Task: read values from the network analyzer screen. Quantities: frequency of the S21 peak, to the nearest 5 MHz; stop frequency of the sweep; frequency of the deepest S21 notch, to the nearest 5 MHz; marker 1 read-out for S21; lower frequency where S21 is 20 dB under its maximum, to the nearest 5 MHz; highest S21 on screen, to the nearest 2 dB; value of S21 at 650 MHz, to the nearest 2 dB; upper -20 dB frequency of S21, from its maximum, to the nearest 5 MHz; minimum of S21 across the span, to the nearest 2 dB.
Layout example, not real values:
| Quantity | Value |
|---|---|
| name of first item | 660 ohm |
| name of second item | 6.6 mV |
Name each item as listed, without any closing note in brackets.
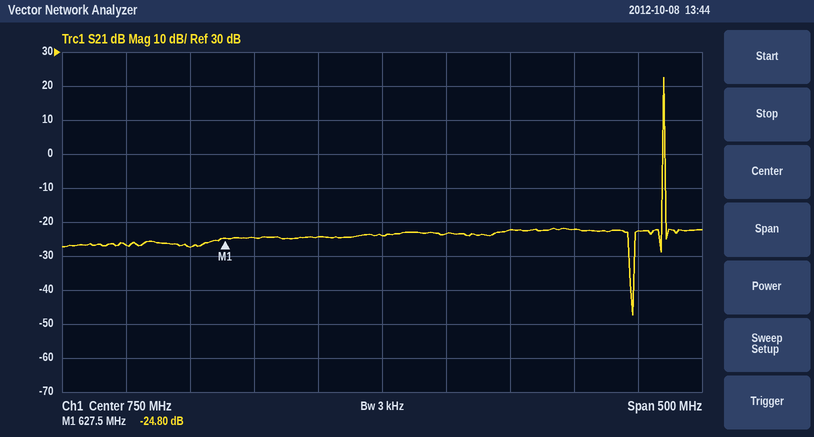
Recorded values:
| Quantity | Value |
|---|---|
| frequency of the S21 peak, to the nearest 5 MHz | 970 MHz |
| stop frequency of the sweep | 1 GHz |
| frequency of the deepest S21 notch, to the nearest 5 MHz | 945 MHz |
| marker 1 read-out for S21 | -24.80 dB |
| lower frequency where S21 is 20 dB under its maximum, to the nearest 5 MHz | 970 MHz |
| highest S21 on screen, to the nearest 2 dB | 22 dB |
| value of S21 at 650 MHz, to the nearest 2 dB | -24 dB |
| upper -20 dB frequency of S21, from its maximum, to the nearest 5 MHz | 970 MHz |
| minimum of S21 across the span, to the nearest 2 dB | -48 dB |
